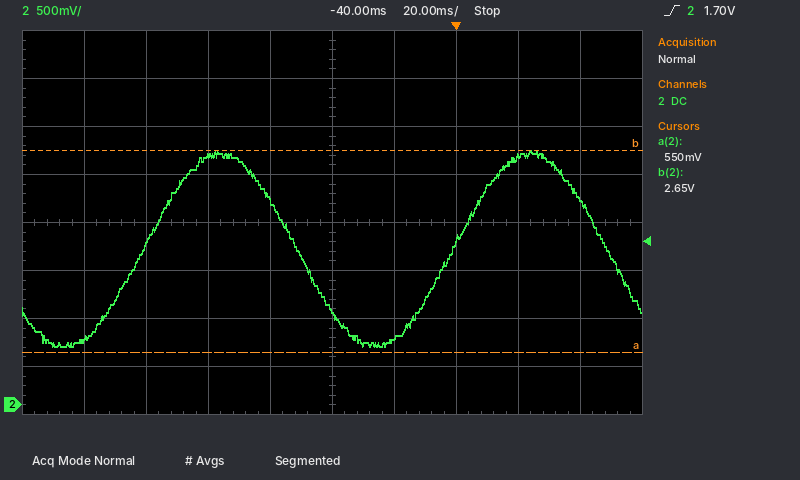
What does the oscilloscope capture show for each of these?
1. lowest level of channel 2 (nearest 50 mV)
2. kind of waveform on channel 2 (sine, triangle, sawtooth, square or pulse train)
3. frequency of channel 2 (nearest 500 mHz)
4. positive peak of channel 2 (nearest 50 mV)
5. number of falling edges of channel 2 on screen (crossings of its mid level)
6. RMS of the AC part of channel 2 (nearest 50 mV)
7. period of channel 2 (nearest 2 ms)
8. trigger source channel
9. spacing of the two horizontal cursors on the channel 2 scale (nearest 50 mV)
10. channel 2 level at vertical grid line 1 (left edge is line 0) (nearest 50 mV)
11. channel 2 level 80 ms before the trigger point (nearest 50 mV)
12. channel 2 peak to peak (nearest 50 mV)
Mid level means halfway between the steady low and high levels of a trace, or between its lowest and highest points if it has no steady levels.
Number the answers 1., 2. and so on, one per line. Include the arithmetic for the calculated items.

1. 600 mV
2. sine
3. 1 / 100 ms ≈ 10.0 Hz
4. 2.65 V
5. 2
6. 2.05 V / (2√2) ≈ 725 mV, so 700 mV to the nearest 50 mV
7. 100 ms
8. channel 2
9. 2.10 V
10. 700 mV
11. 2.60 V
12. 2.65 V − (600 mV) = 2.05 V
